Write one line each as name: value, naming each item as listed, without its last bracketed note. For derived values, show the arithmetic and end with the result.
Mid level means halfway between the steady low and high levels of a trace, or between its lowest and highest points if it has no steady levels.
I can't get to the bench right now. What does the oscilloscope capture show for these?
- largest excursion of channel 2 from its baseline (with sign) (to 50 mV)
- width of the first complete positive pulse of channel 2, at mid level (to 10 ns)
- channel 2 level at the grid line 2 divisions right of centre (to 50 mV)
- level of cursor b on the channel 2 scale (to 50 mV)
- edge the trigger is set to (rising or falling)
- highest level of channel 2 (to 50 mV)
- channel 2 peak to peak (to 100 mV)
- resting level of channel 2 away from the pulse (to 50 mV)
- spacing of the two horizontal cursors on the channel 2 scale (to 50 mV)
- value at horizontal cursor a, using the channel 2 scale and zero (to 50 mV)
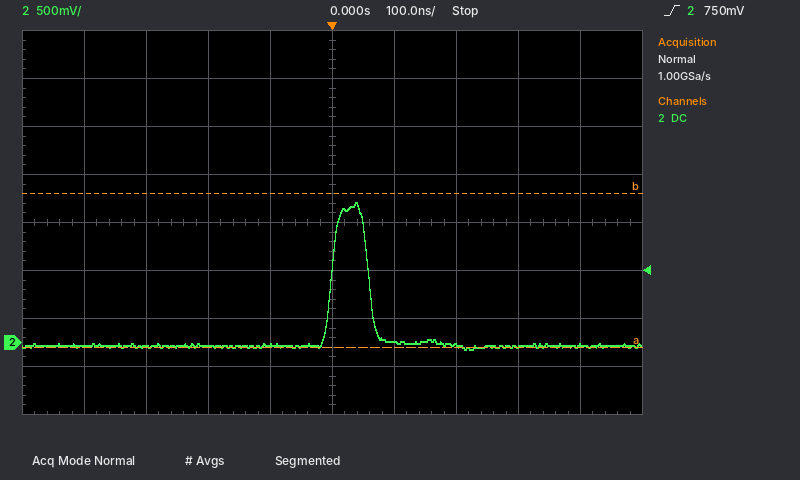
largest excursion of channel 2 from its baseline (with sign): 1.45 V − (-50 mV) = +1.50 V
width of the first complete positive pulse of channel 2, at mid level: 60 ns
channel 2 level at the grid line 2 divisions right of centre: -50 mV
level of cursor b on the channel 2 scale: 1.55 V
edge the trigger is set to: rising
highest level of channel 2: 1.45 V
channel 2 peak to peak: 1.50 V
resting level of channel 2 away from the pulse: -50 mV
spacing of the two horizontal cursors on the channel 2 scale: 1.60 V
value at horizontal cursor a, using the channel 2 scale and zero: -50 mV
